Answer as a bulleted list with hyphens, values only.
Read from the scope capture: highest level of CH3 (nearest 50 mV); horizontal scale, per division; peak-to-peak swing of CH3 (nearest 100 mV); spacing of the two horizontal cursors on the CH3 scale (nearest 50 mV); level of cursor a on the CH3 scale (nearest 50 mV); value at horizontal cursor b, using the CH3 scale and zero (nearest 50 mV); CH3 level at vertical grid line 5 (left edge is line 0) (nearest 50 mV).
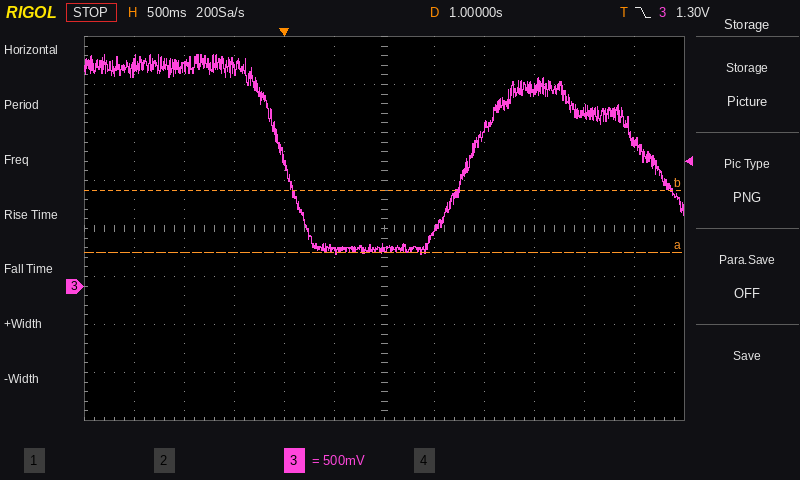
- 2.40 V
- 500 ms
- 2.10 V
- 650 mV
- 350 mV
- 1.00 V
- 350 mV
